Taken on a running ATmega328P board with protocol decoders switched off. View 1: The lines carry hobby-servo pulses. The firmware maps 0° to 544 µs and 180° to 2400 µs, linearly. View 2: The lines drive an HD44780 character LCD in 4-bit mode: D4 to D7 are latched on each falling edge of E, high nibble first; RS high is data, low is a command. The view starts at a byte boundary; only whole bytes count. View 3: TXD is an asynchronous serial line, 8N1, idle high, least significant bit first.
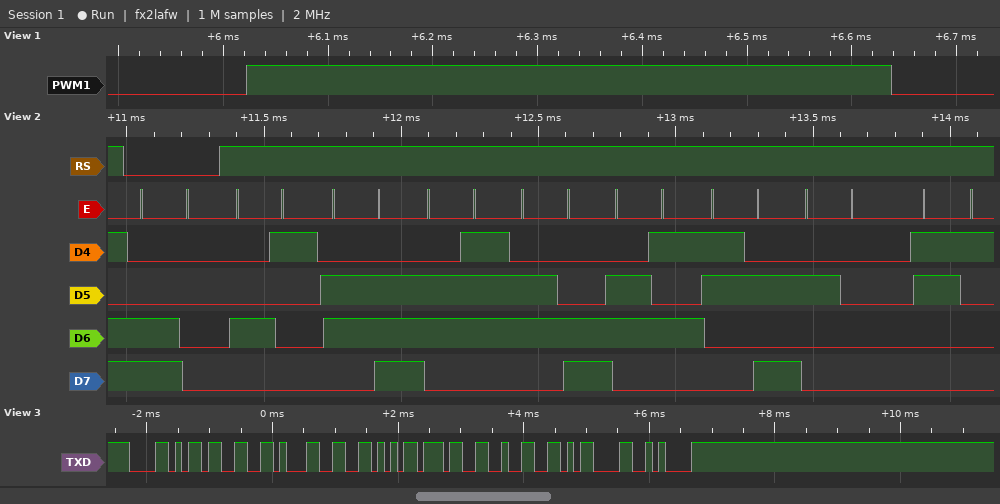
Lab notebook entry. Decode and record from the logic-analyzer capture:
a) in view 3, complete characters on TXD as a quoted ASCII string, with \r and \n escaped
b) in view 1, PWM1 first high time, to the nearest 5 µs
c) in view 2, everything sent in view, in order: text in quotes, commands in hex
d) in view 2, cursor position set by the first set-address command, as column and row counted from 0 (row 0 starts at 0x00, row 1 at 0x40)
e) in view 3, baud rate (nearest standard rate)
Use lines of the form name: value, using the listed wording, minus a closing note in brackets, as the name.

in view 3, complete characters on TXD as a quoted ASCII string, with \r and \n escaped: "X31V72\r\n"
in view 1, PWM1 first high time, to the nearest 5 µs: 615 µs
in view 2, everything sent in view, in order: text in quotes, commands in hex: 0xC0 "Angle: 1"
in view 2, cursor position set by the first set-address command, as column and row counted from 0: column 0, row 1
in view 3, baud rate: 9600 baud
